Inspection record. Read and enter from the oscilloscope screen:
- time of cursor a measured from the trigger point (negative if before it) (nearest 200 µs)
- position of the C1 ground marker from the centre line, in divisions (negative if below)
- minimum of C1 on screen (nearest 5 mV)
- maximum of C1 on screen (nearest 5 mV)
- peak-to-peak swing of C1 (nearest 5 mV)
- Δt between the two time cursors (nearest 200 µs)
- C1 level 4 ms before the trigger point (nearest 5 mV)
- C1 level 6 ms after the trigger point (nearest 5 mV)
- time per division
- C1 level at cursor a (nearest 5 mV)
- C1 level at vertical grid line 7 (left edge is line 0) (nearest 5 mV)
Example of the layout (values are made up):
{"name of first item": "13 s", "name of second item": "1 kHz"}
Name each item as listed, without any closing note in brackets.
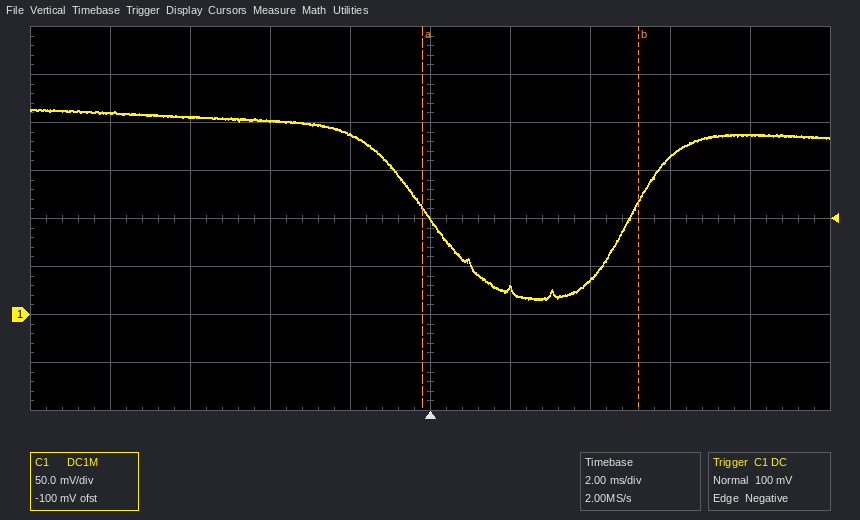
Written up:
{"time of cursor a measured from the trigger point (negative if before it)": "-200 µs", "position of the C1 ground marker from the centre line, in divisions": "-2.0 div", "minimum of C1 on screen": "15 mV", "maximum of C1 on screen": "215 mV", "peak-to-peak swing of C1": "200 mV", "Δt between the two time cursors": "5.4 ms", "C1 level 4 ms before the trigger point": "200 mV", "C1 level 6 ms after the trigger point": "165 mV", "time per division": "2 ms", "C1 level at cursor a": "110 mV", "C1 level at vertical grid line 7 (left edge is line 0)": "35 mV"}
